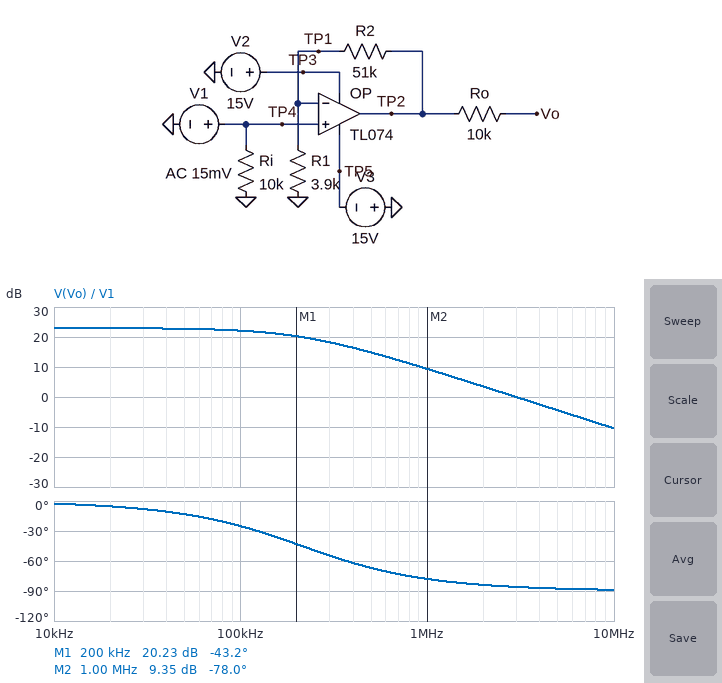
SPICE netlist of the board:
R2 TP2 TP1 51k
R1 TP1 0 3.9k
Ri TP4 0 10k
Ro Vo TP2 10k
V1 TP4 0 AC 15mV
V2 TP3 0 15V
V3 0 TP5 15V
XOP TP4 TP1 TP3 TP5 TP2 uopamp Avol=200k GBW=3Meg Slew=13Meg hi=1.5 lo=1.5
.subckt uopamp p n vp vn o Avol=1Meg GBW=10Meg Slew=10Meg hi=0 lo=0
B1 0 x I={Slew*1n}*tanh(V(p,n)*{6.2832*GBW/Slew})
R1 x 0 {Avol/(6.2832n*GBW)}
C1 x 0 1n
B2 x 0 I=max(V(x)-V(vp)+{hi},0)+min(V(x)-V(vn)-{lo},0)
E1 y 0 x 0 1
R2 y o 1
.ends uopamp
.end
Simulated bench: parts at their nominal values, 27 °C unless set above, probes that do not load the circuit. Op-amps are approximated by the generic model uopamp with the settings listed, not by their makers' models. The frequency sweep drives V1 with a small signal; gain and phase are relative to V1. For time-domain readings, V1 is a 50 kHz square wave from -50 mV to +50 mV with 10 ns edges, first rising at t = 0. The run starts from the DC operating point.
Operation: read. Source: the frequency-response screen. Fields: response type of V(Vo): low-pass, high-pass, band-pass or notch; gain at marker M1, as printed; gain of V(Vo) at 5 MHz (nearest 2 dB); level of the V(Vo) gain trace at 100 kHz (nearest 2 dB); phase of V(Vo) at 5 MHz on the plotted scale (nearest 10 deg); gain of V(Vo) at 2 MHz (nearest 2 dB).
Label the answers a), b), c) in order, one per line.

a) low-pass
b) 20.23 dB
c) -4 dB
d) 22 dB
e) -90 deg
f) 4 dB
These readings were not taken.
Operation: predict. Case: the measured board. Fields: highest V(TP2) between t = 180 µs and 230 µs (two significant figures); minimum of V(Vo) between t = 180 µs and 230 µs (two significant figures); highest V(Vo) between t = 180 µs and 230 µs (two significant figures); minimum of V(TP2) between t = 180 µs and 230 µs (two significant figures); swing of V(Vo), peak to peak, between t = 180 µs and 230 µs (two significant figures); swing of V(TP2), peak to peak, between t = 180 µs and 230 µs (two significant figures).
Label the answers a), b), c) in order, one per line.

a) 700 mV
b) -700 mV
c) 700 mV
d) -700 mV
e) 1.4 V
f) 1.4 V
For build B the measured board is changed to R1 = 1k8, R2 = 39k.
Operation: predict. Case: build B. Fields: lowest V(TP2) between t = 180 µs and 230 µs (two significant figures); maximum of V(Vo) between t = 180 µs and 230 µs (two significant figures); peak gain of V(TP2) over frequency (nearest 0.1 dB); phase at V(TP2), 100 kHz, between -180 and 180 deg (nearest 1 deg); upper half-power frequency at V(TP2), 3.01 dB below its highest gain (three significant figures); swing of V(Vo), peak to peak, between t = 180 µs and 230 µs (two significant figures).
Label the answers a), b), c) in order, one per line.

a) -1.1 V
b) 1.1 V
c) 27.1 dB
d) -37 deg
e) 132 kHz
f) 2.3 V
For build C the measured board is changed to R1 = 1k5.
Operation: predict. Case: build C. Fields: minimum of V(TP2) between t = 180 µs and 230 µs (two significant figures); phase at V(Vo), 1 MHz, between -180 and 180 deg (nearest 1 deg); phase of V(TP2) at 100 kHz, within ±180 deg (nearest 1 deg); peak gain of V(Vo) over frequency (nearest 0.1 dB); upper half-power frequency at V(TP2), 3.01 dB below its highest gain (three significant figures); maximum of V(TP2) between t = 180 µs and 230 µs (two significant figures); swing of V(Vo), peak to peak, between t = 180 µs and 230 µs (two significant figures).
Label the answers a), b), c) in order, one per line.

a) -1.7 V
b) -85 deg
c) -49 deg
d) 30.9 dB
e) 85.7 kHz
f) 1.7 V
g) 3.5 V
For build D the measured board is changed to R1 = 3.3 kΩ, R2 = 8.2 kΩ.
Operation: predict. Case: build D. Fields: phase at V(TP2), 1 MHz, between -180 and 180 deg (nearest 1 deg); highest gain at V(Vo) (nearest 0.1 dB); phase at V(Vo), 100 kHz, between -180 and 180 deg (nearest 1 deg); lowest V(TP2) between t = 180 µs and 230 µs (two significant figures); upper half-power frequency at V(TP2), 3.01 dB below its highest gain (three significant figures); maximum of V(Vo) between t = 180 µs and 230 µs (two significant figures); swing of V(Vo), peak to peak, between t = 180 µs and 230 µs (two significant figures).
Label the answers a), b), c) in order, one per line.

a) -49 deg
b) 10.8 dB
c) -7 deg
d) -170 mV
e) 861 kHz
f) 170 mV
g) 350 mV
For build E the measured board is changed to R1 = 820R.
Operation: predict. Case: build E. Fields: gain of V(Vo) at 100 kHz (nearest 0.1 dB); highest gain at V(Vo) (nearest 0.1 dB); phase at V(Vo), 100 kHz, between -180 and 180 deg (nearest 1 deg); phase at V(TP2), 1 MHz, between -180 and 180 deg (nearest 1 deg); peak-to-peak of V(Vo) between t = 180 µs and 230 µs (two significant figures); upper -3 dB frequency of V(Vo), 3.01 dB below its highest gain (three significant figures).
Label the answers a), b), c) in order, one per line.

a) 28.7 dB
b) 36.0 dB
c) -65 deg
d) -87 deg
e) 5.7 V
f) 47.5 kHz
